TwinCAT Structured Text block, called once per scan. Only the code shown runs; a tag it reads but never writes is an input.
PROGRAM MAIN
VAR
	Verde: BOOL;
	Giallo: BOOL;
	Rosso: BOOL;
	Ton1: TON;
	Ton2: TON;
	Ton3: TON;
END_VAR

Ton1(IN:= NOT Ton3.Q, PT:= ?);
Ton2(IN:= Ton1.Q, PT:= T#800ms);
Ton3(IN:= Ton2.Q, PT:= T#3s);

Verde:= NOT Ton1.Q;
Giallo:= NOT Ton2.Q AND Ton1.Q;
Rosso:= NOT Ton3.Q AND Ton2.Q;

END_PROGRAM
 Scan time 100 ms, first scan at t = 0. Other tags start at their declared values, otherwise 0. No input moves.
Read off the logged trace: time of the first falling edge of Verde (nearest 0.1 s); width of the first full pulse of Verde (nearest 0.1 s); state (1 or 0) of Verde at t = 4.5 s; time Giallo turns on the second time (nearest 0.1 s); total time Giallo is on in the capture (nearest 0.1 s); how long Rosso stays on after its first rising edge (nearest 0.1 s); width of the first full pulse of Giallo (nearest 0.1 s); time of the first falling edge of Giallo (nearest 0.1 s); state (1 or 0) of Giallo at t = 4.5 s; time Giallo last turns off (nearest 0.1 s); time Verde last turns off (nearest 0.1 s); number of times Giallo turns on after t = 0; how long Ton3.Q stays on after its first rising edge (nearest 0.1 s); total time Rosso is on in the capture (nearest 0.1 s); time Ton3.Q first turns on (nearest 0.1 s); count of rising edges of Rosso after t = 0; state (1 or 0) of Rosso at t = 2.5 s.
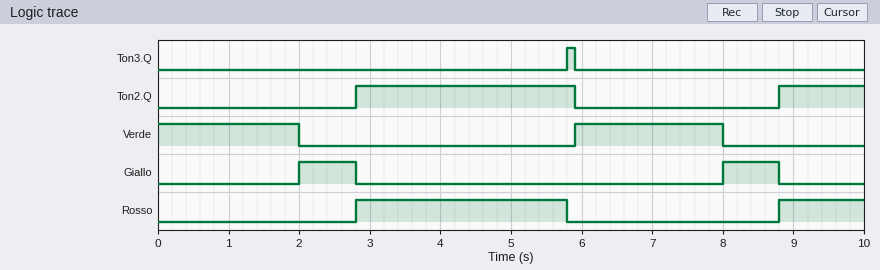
2.0 s
2.1 s
0
8.0 s
1.6 s
3.0 s
0.8 s
2.8 s
0
8.8 s
8.0 s
2
0.1 s
4.2 s
5.8 s
2
0
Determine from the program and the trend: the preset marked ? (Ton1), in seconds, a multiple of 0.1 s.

2.0 s
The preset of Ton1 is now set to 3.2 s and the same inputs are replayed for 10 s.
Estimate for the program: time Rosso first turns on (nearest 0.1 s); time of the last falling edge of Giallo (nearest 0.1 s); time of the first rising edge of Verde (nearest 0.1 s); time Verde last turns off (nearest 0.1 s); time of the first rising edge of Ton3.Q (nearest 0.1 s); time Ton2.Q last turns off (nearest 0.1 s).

4.0 s
4.0 s
7.1 s
3.2 s
7.0 s
7.1 s
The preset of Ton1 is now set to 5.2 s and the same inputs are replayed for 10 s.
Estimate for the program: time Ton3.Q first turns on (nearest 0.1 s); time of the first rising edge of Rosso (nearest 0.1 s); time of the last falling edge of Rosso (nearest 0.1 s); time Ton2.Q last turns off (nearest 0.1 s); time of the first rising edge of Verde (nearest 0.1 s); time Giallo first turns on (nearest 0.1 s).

9.0 s
6.0 s
9.0 s
9.1 s
9.1 s
5.2 s
